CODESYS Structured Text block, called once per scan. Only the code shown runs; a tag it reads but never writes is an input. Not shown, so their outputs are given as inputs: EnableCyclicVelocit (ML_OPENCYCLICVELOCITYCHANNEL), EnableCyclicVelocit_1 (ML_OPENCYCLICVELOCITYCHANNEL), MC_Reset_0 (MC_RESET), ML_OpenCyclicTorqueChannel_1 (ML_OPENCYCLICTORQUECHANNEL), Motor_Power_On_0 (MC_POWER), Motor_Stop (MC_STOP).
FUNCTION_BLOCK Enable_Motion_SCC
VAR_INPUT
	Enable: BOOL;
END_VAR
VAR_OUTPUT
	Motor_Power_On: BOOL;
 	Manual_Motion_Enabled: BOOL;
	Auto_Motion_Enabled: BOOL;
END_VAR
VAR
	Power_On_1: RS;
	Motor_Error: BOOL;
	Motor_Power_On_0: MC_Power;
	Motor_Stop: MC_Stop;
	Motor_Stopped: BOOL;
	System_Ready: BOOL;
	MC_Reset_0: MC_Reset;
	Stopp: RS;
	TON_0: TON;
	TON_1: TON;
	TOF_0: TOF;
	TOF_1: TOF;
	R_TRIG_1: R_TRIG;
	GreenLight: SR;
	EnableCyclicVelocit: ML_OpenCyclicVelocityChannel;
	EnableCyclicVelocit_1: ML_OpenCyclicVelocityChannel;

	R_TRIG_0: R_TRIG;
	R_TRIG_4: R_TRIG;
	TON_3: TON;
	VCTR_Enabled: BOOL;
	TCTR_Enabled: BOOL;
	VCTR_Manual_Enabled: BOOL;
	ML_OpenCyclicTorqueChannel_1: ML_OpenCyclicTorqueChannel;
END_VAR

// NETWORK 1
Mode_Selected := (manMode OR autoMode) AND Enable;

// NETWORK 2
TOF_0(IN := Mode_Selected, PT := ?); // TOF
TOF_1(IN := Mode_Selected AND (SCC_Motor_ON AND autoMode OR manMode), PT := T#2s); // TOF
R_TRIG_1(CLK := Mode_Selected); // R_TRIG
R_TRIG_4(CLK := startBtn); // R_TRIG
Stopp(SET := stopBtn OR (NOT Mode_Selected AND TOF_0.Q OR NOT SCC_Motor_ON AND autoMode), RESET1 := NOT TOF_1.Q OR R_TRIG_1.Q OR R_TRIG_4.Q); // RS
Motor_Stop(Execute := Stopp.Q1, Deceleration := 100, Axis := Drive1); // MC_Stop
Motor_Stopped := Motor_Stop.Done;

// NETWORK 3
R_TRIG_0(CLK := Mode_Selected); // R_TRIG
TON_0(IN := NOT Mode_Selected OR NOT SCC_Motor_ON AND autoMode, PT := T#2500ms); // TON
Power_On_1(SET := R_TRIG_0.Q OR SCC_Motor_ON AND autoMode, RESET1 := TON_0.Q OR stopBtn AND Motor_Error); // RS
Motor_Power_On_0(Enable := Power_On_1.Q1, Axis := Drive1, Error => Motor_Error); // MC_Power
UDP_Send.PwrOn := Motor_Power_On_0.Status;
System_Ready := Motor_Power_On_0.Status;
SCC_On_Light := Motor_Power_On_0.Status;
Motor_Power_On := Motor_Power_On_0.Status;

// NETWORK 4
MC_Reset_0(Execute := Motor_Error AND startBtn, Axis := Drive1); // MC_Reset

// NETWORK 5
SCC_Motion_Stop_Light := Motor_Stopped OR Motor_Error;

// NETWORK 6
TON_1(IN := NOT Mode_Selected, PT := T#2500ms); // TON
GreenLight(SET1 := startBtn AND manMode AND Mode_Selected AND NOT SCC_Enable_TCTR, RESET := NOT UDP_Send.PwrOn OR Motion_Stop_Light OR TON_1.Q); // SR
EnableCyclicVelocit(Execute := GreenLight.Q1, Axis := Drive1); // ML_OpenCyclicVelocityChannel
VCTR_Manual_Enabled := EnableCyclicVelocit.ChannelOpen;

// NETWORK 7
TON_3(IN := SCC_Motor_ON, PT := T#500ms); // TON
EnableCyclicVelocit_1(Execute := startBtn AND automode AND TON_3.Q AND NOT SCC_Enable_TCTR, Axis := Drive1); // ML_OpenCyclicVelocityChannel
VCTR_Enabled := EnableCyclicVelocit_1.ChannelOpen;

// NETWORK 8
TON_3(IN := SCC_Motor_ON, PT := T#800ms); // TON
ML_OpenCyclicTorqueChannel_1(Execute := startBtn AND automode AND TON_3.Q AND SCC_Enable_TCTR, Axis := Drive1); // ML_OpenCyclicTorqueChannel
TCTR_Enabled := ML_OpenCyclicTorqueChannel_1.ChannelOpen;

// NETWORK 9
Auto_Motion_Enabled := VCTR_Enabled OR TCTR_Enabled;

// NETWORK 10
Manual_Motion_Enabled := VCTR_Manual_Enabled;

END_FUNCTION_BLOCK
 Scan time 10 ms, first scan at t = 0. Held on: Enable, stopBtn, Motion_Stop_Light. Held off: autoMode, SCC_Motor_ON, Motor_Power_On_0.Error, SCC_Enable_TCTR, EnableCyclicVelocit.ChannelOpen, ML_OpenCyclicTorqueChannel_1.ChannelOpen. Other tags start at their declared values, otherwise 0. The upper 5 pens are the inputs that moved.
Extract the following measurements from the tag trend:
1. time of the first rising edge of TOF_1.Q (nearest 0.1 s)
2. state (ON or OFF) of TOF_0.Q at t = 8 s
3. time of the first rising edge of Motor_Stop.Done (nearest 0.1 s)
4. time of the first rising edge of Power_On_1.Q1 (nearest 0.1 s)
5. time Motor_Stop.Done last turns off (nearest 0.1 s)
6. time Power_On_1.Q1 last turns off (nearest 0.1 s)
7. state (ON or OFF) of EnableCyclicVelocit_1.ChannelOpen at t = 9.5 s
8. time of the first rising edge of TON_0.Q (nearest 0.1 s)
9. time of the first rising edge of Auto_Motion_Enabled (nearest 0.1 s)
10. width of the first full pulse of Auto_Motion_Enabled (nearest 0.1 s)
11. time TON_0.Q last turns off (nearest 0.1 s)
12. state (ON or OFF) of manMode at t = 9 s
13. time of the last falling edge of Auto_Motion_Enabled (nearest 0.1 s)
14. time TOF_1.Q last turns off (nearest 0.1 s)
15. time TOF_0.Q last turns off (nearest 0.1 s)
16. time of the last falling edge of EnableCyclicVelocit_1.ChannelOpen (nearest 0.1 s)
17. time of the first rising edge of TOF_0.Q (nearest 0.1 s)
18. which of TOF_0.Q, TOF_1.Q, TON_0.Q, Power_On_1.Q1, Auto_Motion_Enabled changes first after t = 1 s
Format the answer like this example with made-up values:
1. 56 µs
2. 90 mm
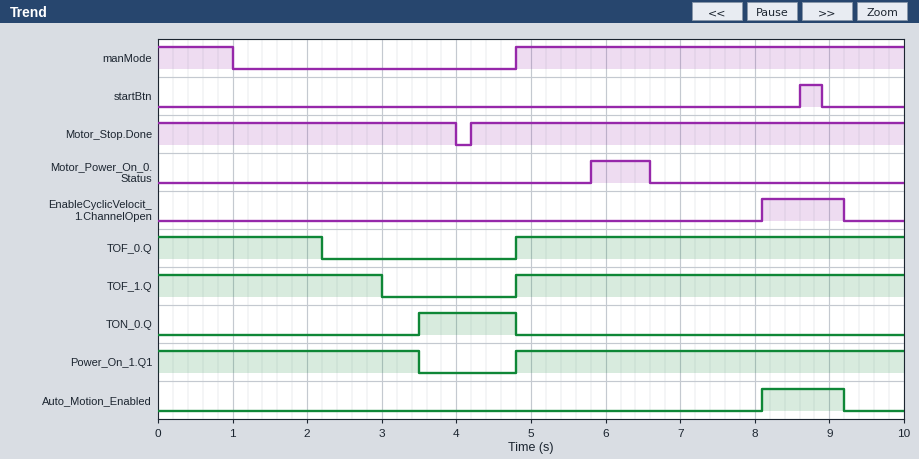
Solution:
1. 4.8 s
2. ON
3. 4.2 s
4. 4.8 s
5. 4.0 s
6. 3.5 s
7. OFF
8. 3.5 s
9. 8.1 s
10. 1.1 s
11. 4.8 s
12. ON
13. 9.2 s
14. 3.0 s
15. 2.2 s
16. 9.2 s
17. 4.8 s
18. TOF_0.Q
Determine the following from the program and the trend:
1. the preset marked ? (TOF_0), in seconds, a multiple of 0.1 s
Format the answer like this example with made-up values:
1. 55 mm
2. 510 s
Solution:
1. 1.2 s
